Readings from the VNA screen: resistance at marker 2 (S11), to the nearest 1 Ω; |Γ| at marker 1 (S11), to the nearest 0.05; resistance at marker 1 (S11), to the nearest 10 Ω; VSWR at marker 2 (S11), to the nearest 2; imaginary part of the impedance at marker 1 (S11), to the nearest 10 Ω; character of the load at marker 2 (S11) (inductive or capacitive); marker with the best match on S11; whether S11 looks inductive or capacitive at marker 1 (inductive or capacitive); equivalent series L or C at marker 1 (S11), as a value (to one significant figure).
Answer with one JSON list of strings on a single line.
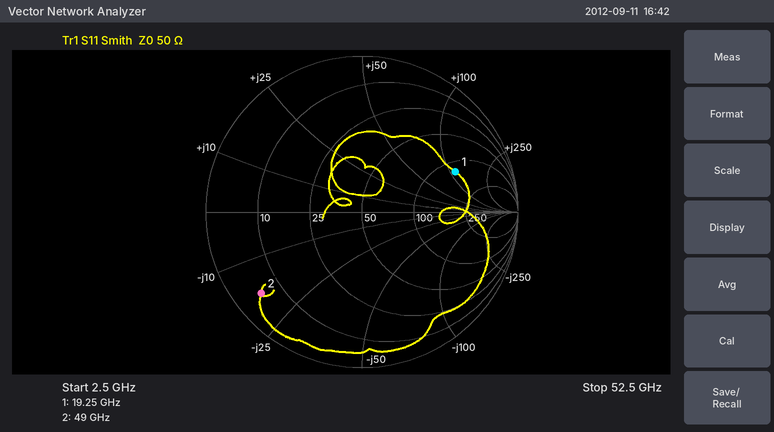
["5 Ω", "0.65", "130 Ω", "10", "+110 Ω", "capacitive", "marker 1", "inductive", "900 pH"]
